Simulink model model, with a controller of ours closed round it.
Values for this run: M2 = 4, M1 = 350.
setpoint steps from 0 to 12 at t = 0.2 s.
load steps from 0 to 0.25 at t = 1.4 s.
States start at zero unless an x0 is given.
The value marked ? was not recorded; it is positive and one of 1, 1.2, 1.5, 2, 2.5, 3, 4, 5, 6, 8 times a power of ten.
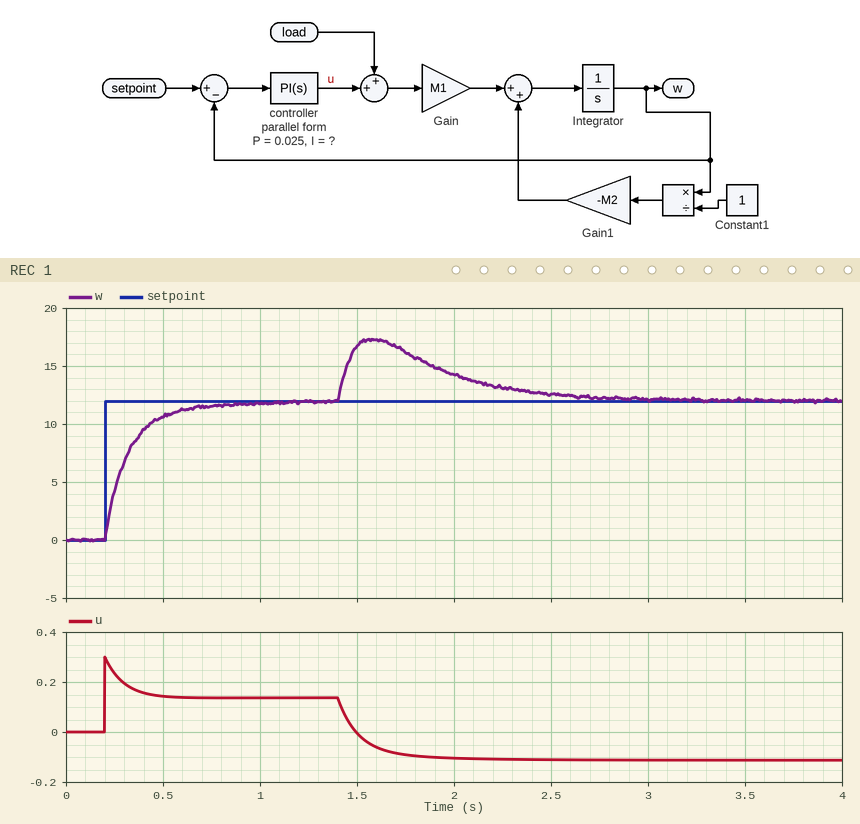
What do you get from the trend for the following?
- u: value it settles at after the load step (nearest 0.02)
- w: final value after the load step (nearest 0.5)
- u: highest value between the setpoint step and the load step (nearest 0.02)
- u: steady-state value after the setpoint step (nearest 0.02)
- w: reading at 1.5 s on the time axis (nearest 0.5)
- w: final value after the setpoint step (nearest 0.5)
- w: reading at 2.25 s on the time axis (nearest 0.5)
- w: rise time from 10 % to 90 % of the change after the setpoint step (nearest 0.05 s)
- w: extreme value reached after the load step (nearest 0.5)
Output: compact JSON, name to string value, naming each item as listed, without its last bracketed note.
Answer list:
{"u: value it settles at after the load step": "-0.12", "w: final value after the load step": "12.0", "u: highest value between the setpoint step and the load step": "0.30", "u: steady-state value after the setpoint step": "0.14", "w: reading at 1.5 s on the time axis": "16.5", "w: final value after the setpoint step": "12.0", "w: reading at 2.25 s on the time axis": "13.0", "w: rise time from 10 % to 90 % of the change after the setpoint step": "0.30 s", "w: extreme value reached after the load step": "17.5"}
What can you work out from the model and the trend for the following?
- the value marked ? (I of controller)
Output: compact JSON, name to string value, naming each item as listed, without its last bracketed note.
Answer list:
{"the value marked ?": "0.08"}
